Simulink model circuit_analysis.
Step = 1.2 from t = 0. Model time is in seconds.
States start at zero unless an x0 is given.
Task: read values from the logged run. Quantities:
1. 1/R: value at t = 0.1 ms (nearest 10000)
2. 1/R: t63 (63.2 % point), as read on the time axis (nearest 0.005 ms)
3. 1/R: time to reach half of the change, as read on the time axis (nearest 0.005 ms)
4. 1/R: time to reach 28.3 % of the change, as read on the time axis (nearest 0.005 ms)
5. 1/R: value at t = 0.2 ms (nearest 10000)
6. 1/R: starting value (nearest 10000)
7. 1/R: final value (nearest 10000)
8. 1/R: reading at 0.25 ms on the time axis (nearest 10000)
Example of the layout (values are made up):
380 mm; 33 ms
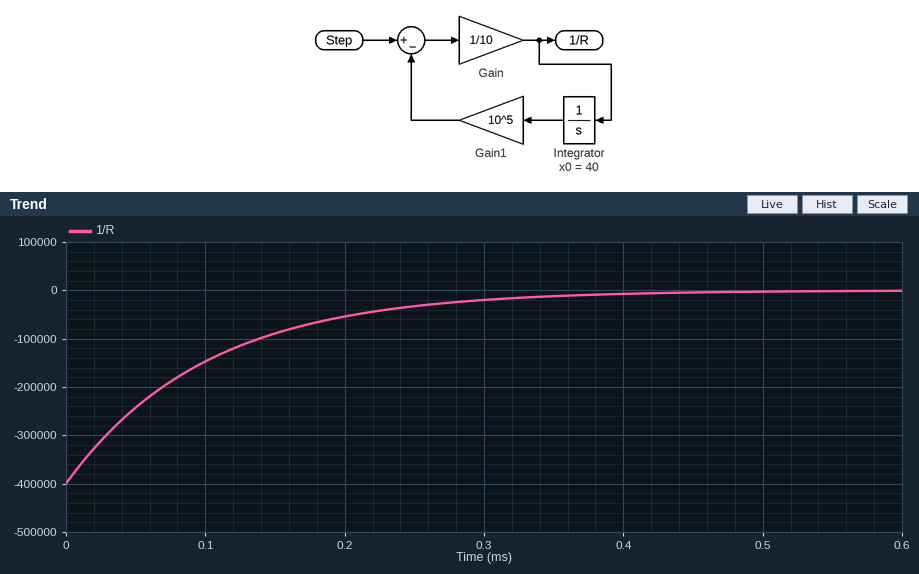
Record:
-150000; 0.100 ms; 0.070 ms; 0.035 ms; -50000; -400000; 0; -30000
